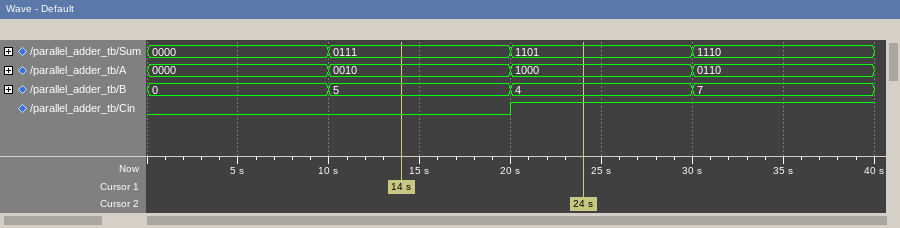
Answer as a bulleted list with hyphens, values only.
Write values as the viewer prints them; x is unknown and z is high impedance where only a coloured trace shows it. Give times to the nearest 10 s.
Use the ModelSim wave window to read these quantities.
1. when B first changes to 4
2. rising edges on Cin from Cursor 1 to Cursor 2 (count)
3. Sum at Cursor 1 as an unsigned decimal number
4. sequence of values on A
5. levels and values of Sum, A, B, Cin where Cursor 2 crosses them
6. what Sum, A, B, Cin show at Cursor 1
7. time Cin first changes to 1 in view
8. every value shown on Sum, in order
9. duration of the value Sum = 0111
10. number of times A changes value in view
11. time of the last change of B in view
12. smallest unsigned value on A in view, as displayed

- 20 s
- 1
- 7
- 0000, 0010, 1000, 0110
- Sum=1101, A=1000, B=4, Cin=1
- Sum=0111, A=0010, B=5, Cin=0
- 20 s
- 0000, 0111, 1101, 1110
- 10 s
- 3
- 30 s
- 0000
